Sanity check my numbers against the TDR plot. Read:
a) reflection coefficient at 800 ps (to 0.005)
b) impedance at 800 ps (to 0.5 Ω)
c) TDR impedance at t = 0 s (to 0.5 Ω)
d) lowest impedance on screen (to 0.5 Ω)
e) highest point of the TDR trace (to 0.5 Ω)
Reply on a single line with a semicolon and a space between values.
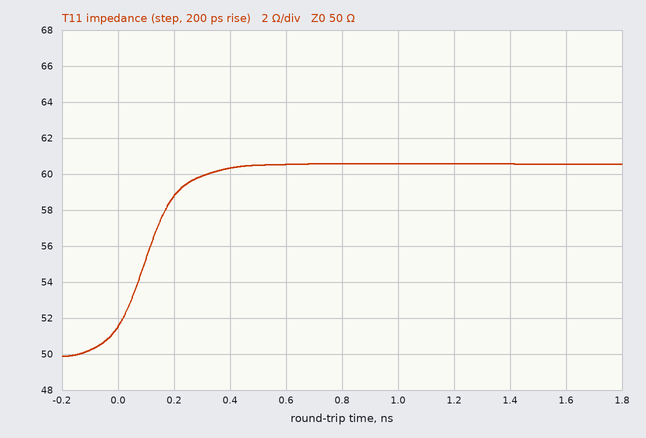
+0.095; 60.5 Ω; 51.5 Ω; 50.0 Ω; 60.5 Ω
